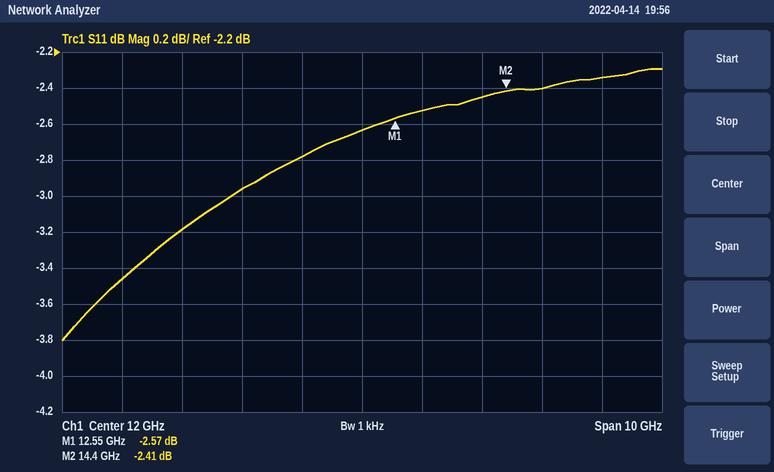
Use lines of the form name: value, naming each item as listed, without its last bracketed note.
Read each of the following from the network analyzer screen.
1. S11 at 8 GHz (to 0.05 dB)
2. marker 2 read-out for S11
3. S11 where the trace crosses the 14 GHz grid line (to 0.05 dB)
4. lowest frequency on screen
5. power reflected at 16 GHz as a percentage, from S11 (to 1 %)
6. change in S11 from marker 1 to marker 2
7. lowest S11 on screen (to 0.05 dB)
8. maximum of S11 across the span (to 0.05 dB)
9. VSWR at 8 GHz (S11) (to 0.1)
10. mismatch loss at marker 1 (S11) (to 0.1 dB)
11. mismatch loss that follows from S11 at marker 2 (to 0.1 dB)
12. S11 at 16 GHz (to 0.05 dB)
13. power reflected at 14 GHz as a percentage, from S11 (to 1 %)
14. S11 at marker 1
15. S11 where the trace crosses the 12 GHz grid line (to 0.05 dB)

S11 at 8 GHz: -3.45 dB
marker 2 read-out for S11: -2.41 dB
S11 where the trace crosses the 14 GHz grid line: -2.45 dB
lowest frequency on screen: 7 GHz
power reflected at 16 GHz as a percentage, from S11: 58 %
change in S11 from marker 1 to marker 2: 0.16 dB
lowest S11 on screen: -3.80 dB
maximum of S11 across the span: -2.30 dB
VSWR at 8 GHz (S11): 5.1
mismatch loss at marker 1 (S11): 3.5 dB
mismatch loss that follows from S11 at marker 2: 3.7 dB
S11 at 16 GHz: -2.35 dB
power reflected at 14 GHz as a percentage, from S11: 57 %
S11 at marker 1: -2.57 dB
S11 where the trace crosses the 12 GHz grid line: -2.65 dB
